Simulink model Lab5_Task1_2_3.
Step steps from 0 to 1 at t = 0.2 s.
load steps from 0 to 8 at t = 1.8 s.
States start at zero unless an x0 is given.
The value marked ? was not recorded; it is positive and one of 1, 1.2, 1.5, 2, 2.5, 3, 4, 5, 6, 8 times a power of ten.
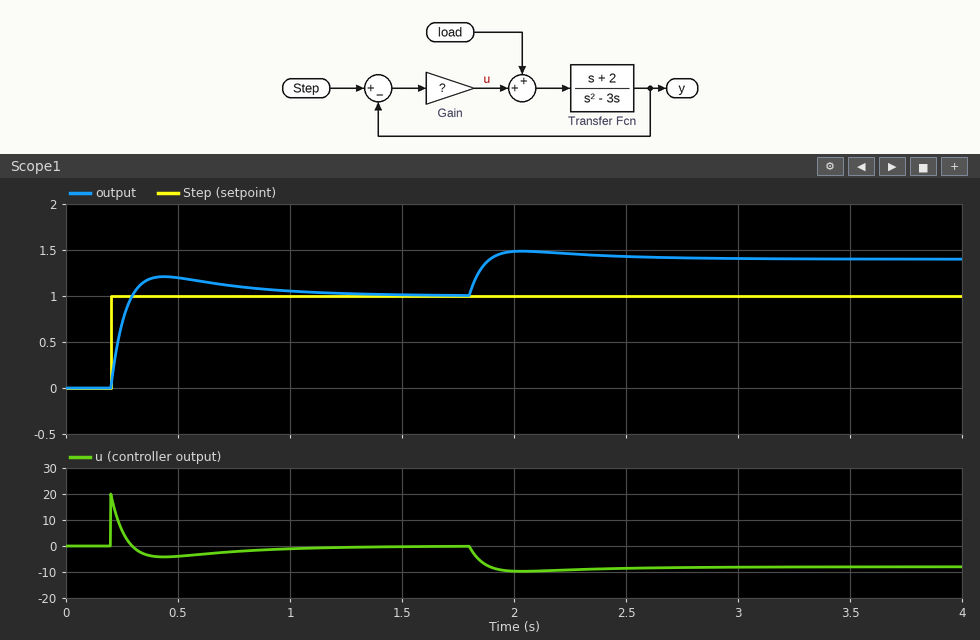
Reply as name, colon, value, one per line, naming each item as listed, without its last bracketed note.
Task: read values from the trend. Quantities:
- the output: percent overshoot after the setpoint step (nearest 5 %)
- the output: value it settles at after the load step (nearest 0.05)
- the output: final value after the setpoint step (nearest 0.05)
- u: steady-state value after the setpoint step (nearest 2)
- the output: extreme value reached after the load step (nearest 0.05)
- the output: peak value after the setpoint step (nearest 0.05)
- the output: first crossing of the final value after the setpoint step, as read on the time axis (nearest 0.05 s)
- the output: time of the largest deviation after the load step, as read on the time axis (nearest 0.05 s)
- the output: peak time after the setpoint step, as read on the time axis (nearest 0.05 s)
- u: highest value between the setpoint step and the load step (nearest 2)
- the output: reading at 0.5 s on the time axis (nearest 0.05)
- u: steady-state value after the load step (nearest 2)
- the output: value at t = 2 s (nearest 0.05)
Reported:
the output: percent overshoot after the setpoint step: 20 %
the output: value it settles at after the load step: 1.40
the output: final value after the setpoint step: 1.00
u: steady-state value after the setpoint step: 0
the output: extreme value reached after the load step: 1.50
the output: peak value after the setpoint step: 1.20
the output: first crossing of the final value after the setpoint step, as read on the time axis: 0.30 s
the output: time of the largest deviation after the load step, as read on the time axis: 2.05 s
the output: peak time after the setpoint step, as read on the time axis: 0.45 s
u: highest value between the setpoint step and the load step: 20
the output: reading at 0.5 s on the time axis: 1.20
u: steady-state value after the load step: -8
the output: value at t = 2 s: 1.50
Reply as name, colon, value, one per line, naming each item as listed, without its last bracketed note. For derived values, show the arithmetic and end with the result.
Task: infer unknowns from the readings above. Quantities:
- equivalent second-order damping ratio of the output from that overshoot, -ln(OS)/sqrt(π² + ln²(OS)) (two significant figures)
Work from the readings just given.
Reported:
equivalent second-order damping ratio of the output from that overshoot, -ln(OS)/sqrt(π² + ln²(OS)): ln(0.2) = -1.609; 1.609 / sqrt(9.870 + 2.590) = 0.46
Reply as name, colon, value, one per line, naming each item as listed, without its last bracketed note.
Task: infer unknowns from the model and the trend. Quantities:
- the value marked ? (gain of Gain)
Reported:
the value marked ?: 20
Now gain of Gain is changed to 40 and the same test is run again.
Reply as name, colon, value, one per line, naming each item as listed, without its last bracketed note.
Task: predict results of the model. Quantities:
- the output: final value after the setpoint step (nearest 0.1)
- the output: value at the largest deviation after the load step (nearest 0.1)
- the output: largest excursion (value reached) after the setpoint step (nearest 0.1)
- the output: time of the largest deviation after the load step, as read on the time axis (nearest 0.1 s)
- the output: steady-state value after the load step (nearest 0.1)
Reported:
the output: final value after the setpoint step: 1.0
the output: value at the largest deviation after the load step: 1.2
the output: largest excursion (value reached) after the setpoint step: 1.1
the output: time of the largest deviation after the load step, as read on the time axis: 1.9 s
the output: steady-state value after the load step: 1.2
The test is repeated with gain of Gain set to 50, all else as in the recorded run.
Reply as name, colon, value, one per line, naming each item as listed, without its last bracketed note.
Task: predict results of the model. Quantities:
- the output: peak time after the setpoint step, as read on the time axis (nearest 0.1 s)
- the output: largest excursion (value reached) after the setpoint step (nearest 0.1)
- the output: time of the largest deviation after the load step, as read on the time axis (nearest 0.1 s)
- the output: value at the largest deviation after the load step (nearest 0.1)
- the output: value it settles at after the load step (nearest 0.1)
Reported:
the output: peak time after the setpoint step, as read on the time axis: 0.3 s
the output: largest excursion (value reached) after the setpoint step: 1.1
the output: time of the largest deviation after the load step, as read on the time axis: 1.9 s
the output: value at the largest deviation after the load step: 1.2
the output: value it settles at after the load step: 1.2
